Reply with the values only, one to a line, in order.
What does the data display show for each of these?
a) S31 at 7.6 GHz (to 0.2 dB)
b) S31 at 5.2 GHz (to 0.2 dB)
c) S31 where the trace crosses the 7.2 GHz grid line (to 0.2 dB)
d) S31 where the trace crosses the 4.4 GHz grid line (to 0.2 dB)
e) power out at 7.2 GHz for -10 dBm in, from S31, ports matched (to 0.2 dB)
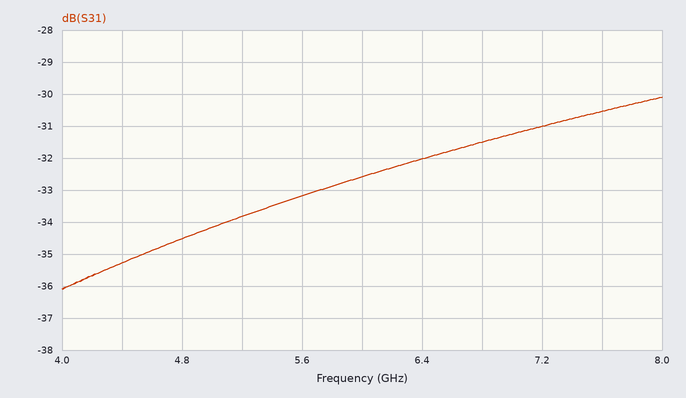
-30.6 dB
-33.8 dB
-31.0 dB
-35.2 dB
-41.0 dBm
